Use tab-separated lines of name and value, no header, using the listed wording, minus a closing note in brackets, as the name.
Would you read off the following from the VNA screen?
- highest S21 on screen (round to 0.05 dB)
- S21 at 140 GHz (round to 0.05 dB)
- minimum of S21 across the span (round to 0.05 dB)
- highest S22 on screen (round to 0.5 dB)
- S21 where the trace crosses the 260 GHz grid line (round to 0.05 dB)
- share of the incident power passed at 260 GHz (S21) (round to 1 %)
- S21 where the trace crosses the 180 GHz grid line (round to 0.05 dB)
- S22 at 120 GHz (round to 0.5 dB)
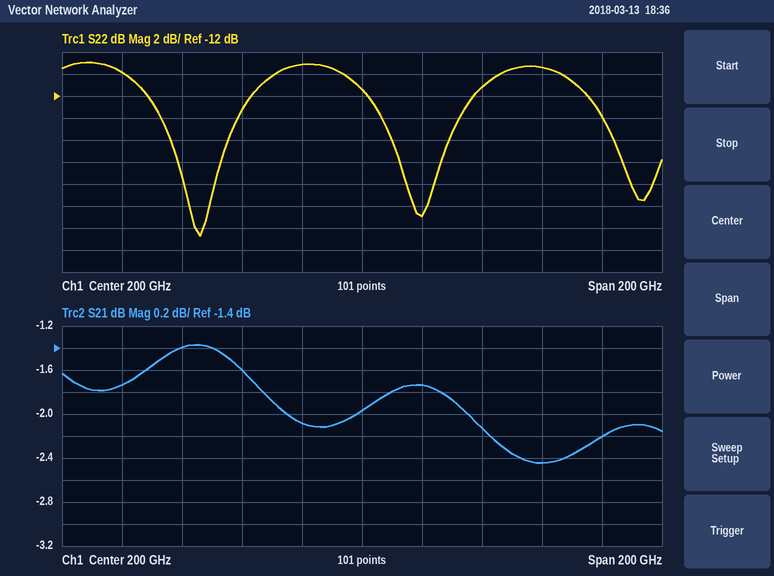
highest S21 on screen	-1.35 dB
S21 at 140 GHz	-1.40 dB
minimum of S21 across the span	-2.45 dB
highest S22 on screen	-9.0 dB
S21 where the trace crosses the 260 GHz grid line	-2.45 dB
share of the incident power passed at 260 GHz (S21)	57 %
S21 where the trace crosses the 180 GHz grid line	-2.10 dB
S22 at 120 GHz	-10.0 dB
